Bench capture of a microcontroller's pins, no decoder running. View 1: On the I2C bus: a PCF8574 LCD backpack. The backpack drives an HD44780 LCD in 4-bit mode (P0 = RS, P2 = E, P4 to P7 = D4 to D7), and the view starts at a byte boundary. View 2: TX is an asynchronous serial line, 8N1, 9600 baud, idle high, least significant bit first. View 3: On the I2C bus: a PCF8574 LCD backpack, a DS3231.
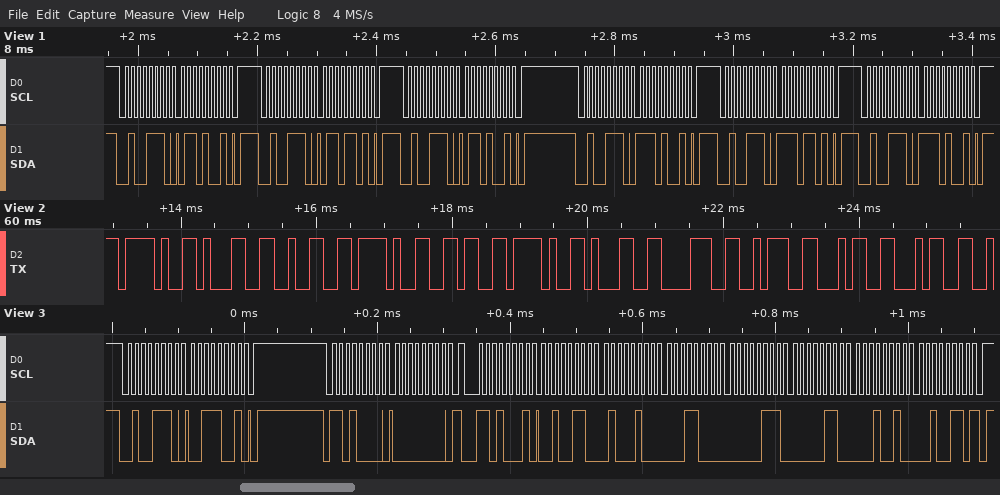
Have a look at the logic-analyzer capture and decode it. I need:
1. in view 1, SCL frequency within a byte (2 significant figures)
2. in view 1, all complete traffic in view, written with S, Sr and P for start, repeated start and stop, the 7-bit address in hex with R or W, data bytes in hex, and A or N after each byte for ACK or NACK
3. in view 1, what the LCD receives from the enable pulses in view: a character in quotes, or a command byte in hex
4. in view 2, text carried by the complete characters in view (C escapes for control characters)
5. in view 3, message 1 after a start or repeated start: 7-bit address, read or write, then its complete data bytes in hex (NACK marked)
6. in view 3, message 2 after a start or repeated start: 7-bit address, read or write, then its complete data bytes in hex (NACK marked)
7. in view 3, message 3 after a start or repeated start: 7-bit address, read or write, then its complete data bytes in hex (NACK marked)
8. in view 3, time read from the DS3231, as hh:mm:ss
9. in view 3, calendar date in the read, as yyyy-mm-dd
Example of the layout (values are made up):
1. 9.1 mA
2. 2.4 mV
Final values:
1. 100 kHz
2. S 27W A 69 A P S 27W A 6D A P S 27W A 69 A P S 27W A E9 A P S 27W A ED A P S 27W A E9 A P
3. 'n'
4. "/12/6/18:44"
5. 0x27 write: 39
6. 0x68 write: 00
7. 0x68 read: 26 44 18 07 06 12 26 NACK
8. 18:44:26
9. 2026-12-06
